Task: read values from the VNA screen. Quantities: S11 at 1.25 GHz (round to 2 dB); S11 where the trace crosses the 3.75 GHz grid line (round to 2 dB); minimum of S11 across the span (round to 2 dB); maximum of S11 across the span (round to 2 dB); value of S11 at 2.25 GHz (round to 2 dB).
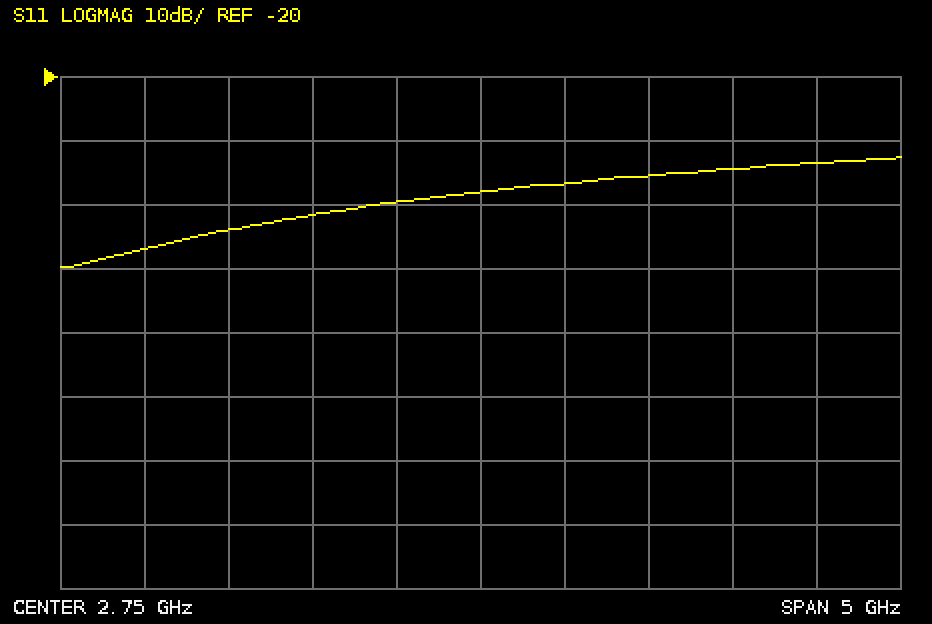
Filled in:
-44 dB
-36 dB
-50 dB
-32 dB
-40 dB
